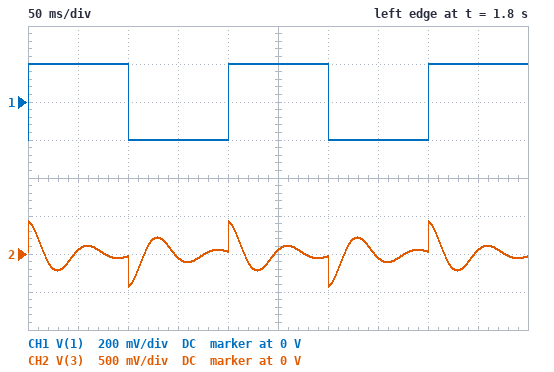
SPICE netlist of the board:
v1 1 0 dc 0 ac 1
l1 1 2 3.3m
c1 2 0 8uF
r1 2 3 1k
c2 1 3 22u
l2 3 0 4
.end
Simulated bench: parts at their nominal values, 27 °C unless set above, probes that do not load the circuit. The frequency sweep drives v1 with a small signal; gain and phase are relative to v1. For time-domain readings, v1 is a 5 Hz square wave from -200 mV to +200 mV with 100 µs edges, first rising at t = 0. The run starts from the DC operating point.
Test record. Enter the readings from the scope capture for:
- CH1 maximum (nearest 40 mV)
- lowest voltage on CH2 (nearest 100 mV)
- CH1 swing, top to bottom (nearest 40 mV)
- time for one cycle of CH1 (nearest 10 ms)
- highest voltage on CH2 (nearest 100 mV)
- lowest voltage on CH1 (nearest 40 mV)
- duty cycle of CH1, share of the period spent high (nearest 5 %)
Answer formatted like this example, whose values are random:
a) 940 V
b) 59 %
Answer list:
a) 200 mV
b) -400 mV
c) 400 mV
d) 200 ms
e) 400 mV
f) -200 mV
g) 50 %
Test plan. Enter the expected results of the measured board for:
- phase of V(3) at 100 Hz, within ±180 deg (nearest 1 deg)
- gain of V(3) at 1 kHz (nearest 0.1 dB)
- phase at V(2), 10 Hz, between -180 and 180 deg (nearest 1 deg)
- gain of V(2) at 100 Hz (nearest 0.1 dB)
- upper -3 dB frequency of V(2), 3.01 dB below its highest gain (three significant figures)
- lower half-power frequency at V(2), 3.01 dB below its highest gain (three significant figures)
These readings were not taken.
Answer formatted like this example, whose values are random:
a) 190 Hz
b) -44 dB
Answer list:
a) 0 deg
b) -0.5 dB
c) 0 deg
d) 0.1 dB
e) 989 Hz
f) 969 Hz
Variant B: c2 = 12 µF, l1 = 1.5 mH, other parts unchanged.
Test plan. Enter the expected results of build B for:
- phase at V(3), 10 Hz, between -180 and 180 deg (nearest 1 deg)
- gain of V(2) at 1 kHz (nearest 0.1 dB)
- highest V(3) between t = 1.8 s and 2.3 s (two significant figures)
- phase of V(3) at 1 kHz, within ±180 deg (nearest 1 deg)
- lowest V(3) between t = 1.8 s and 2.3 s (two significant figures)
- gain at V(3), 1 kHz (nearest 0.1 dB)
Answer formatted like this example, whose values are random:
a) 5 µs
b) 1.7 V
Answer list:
a) 110 deg
b) 5.6 dB
c) 400 mV
d) -1 deg
e) -400 mV
f) 0 dB
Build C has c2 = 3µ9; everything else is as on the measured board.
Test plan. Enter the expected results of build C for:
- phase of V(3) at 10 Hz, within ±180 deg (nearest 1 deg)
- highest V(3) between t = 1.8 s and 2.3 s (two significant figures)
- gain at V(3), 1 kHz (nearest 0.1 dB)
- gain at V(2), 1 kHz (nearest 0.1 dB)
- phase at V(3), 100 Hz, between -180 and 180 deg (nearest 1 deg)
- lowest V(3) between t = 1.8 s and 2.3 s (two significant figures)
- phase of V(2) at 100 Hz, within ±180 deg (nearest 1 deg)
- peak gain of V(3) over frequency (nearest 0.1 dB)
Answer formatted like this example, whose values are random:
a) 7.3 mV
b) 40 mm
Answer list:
a) 89 deg
b) 410 mV
c) -0.2 dB
d) 26.4 dB
e) 4 deg
f) -410 mV
g) 0 deg
h) 3.3 dB
